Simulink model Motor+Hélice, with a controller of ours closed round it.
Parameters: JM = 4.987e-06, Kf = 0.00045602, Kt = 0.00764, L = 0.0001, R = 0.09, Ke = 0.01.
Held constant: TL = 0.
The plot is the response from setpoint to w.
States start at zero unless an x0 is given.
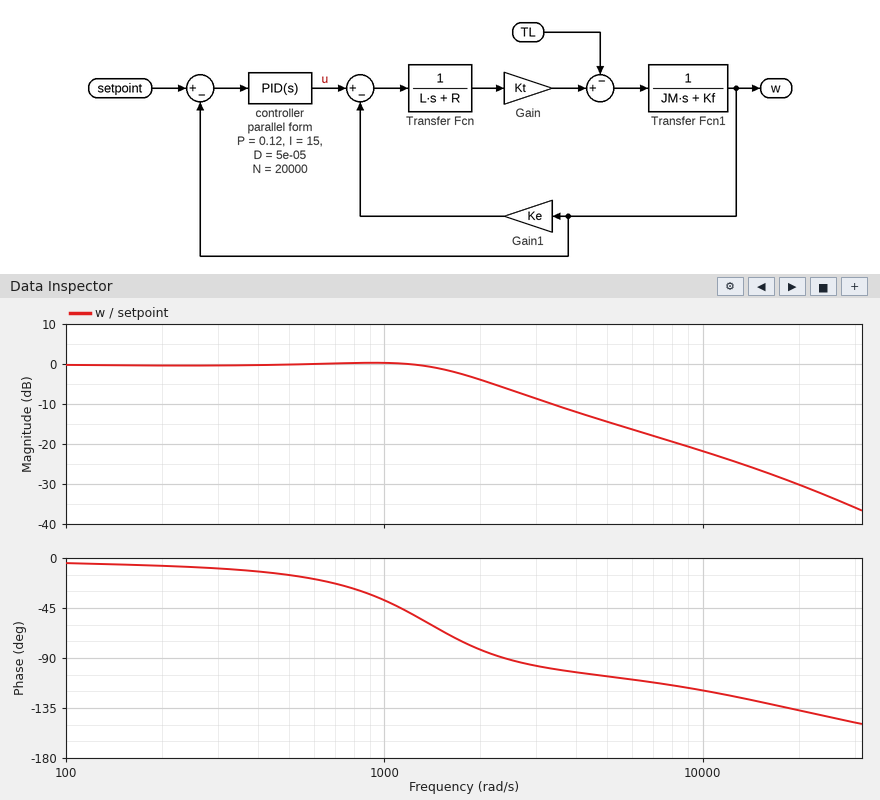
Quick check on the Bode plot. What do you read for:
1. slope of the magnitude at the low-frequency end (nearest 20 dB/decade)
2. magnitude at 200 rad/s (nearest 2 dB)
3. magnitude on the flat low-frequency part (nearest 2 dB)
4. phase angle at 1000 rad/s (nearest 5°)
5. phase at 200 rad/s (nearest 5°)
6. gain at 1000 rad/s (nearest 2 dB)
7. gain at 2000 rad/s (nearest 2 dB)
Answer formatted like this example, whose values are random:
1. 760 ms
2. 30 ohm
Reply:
1. 0 dB/decade
2. 0 dB
3. 0 dB
4. -40°
5. -5°
6. 0 dB
7. -4 dB
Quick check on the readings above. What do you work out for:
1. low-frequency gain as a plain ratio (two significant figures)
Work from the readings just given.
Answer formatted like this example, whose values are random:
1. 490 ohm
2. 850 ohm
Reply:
1. 1.0
